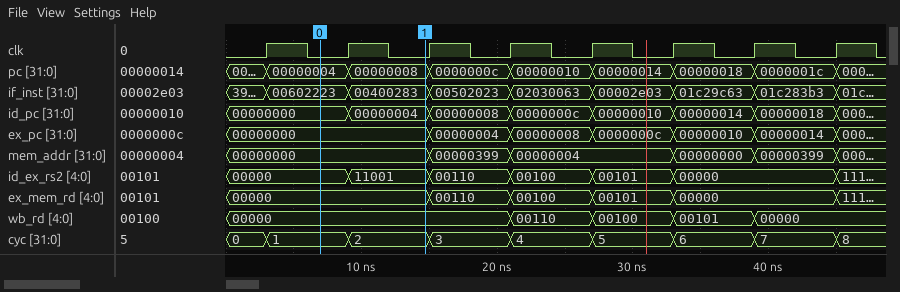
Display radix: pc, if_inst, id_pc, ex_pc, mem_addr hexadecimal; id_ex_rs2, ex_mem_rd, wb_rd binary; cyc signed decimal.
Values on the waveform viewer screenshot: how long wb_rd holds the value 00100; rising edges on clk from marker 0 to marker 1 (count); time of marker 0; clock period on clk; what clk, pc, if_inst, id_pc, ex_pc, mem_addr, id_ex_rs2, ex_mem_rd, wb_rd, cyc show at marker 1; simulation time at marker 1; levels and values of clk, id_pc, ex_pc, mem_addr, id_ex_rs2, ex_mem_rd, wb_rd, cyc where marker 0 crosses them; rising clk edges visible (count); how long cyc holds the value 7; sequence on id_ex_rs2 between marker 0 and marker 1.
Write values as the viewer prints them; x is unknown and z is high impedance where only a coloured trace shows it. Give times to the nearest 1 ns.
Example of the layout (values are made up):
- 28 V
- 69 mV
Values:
- 6 ns
- 1
- 7 ns
- 6 ns
- clk=0, pc=00000008, if_inst=00400283, id_pc=00000004, ex_pc=00000000, mem_addr=00000000, id_ex_rs2=11001, ex_mem_rd=00000, wb_rd=00000, cyc=2
- 15 ns
- clk=0, id_pc=00000000, ex_pc=00000000, mem_addr=00000000, id_ex_rs2=00000, ex_mem_rd=00000, wb_rd=00000, cyc=1
- 8
- 6 ns
- 00000, 11001
